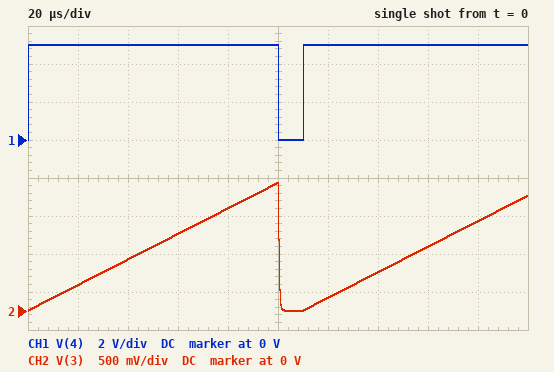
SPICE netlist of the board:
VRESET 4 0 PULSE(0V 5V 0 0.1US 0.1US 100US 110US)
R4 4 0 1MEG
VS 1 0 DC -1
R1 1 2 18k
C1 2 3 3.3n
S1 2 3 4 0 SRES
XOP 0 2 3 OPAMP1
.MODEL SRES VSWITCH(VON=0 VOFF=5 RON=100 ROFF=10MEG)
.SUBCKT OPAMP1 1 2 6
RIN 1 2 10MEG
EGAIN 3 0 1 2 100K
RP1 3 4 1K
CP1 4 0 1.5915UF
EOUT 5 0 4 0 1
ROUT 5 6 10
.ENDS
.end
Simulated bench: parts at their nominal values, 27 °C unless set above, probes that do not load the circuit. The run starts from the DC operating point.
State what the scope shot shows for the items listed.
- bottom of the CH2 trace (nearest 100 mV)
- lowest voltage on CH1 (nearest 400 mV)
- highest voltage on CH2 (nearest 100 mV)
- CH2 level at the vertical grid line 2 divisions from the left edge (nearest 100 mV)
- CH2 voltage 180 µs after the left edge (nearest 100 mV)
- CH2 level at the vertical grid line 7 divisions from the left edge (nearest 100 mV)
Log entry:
0 V
0 V
1.7 V
700 mV
1.2 V
500 mV
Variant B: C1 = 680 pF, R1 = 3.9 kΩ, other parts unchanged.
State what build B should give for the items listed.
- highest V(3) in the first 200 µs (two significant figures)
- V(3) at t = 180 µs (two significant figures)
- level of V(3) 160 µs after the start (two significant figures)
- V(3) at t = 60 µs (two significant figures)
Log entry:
37 V
26 V
19 V
22 V
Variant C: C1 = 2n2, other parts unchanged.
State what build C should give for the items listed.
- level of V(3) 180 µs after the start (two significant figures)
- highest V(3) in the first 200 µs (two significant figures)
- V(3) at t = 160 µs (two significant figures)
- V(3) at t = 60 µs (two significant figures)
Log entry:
1.8 V
2.5 V
1.3 V
1.5 V
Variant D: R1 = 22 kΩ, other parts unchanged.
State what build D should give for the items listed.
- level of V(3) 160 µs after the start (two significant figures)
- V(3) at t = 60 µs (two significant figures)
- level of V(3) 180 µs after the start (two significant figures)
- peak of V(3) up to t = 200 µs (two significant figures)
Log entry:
690 mV
830 mV
970 mV
1.4 V
